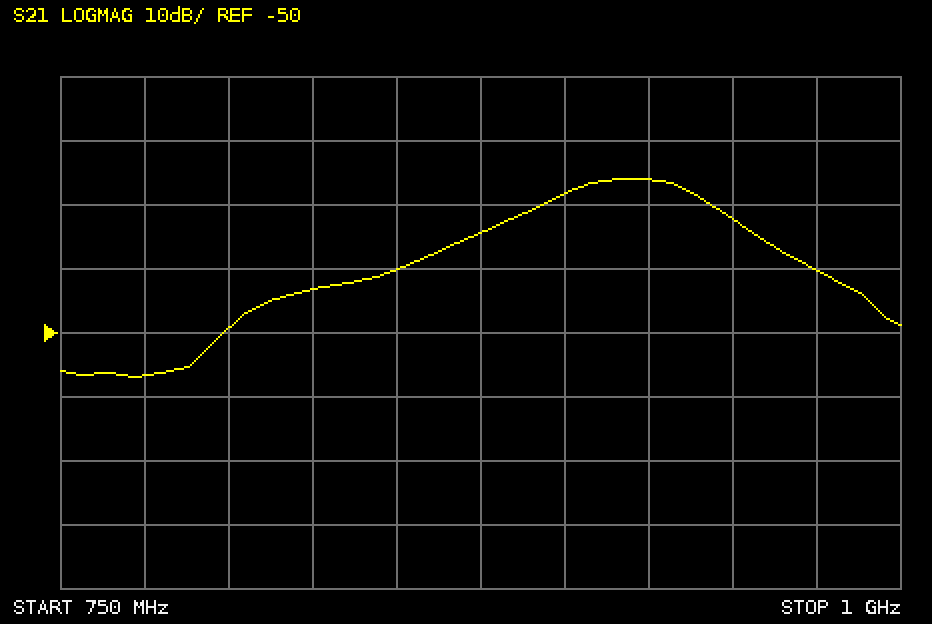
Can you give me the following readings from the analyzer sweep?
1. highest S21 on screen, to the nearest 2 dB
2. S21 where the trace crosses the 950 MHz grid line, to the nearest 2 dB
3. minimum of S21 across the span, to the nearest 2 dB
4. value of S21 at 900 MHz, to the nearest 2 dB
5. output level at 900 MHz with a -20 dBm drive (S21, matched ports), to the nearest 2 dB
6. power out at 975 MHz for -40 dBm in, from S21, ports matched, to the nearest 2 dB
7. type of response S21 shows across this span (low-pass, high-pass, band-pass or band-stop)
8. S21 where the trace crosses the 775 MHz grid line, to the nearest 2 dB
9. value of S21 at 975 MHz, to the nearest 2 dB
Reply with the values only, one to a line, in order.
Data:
-26 dB
-32 dB
-56 dB
-28 dB
-48 dBm
-80 dBm
band-pass
-56 dB
-40 dB
